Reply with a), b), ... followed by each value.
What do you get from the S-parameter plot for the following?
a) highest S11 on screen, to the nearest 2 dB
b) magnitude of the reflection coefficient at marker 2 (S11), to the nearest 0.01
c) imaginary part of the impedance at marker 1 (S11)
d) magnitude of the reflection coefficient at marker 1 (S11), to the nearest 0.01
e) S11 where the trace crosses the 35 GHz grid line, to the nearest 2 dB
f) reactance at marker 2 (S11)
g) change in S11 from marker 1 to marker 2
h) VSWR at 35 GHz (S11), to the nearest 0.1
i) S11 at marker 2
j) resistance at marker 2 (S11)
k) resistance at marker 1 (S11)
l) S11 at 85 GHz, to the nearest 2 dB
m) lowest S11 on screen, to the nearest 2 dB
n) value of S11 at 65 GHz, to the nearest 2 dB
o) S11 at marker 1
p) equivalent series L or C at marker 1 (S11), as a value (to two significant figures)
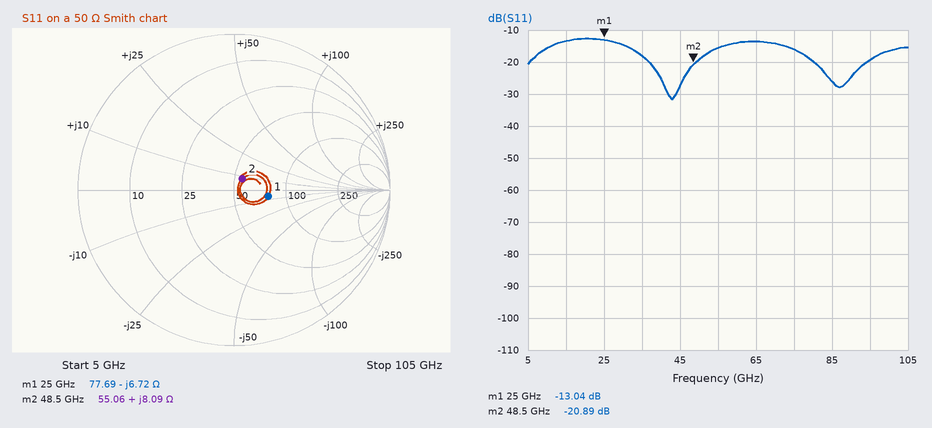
a) -12 dB
b) 0.09
c) -6.72 Ω
d) 0.22
e) -18 dB
f) +8.09 Ω
g) -7.85 dB
h) 1.3
i) -20.89 dB
j) 55.06 Ω
k) 77.69 Ω
l) -26 dB
m) -32 dB
n) -14 dB
o) -13.04 dB
p) 950 fF
